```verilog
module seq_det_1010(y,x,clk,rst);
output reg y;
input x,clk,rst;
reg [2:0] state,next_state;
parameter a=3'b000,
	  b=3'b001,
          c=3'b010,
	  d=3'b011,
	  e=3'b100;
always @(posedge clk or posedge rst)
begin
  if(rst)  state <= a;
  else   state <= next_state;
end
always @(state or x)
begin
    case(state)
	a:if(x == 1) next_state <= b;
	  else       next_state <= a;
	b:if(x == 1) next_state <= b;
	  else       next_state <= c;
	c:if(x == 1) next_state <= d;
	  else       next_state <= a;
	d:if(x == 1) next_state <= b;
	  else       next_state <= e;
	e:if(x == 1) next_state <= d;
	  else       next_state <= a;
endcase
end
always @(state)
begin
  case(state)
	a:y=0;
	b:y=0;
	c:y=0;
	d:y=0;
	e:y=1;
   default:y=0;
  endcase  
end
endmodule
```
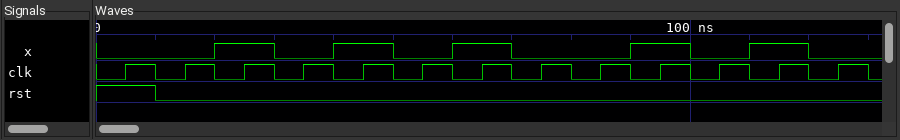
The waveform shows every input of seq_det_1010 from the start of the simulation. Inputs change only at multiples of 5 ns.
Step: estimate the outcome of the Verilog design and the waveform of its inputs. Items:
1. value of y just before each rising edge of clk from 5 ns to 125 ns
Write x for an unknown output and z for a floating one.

0 0 0 0 0 0 1 0 1 0 0 0 0
